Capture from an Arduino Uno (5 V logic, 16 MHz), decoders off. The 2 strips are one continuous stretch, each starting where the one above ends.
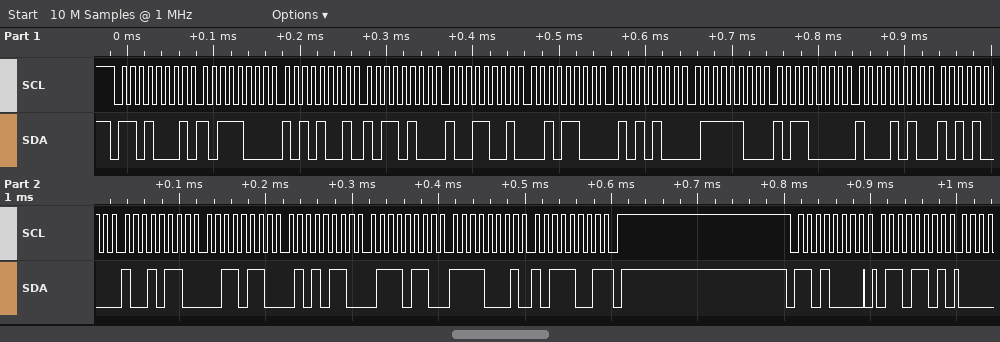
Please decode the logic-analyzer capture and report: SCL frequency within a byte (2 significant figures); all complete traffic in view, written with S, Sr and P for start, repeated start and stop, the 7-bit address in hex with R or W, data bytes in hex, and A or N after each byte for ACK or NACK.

100 kHz
S 68R A B8 A A9 A B4 A 99 A 2C A 54 A 7C A B0 A 8A A A8 A 96 A 36 A 56 A 76 A F1 A B9 N P S 68W A 6D A
